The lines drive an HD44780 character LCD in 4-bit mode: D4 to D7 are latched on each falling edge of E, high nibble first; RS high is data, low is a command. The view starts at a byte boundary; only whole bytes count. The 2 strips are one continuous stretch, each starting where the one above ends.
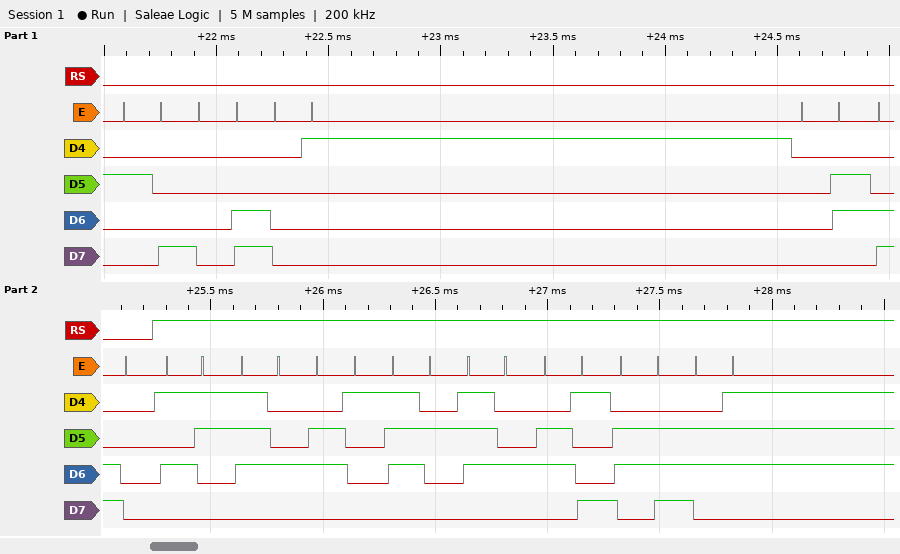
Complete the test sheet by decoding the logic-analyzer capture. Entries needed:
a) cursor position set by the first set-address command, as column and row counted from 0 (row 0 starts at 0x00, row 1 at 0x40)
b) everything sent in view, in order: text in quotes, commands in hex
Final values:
column 0, row 1
0x28 0x0C 0x01 0x06 0xC0 "Starting"
